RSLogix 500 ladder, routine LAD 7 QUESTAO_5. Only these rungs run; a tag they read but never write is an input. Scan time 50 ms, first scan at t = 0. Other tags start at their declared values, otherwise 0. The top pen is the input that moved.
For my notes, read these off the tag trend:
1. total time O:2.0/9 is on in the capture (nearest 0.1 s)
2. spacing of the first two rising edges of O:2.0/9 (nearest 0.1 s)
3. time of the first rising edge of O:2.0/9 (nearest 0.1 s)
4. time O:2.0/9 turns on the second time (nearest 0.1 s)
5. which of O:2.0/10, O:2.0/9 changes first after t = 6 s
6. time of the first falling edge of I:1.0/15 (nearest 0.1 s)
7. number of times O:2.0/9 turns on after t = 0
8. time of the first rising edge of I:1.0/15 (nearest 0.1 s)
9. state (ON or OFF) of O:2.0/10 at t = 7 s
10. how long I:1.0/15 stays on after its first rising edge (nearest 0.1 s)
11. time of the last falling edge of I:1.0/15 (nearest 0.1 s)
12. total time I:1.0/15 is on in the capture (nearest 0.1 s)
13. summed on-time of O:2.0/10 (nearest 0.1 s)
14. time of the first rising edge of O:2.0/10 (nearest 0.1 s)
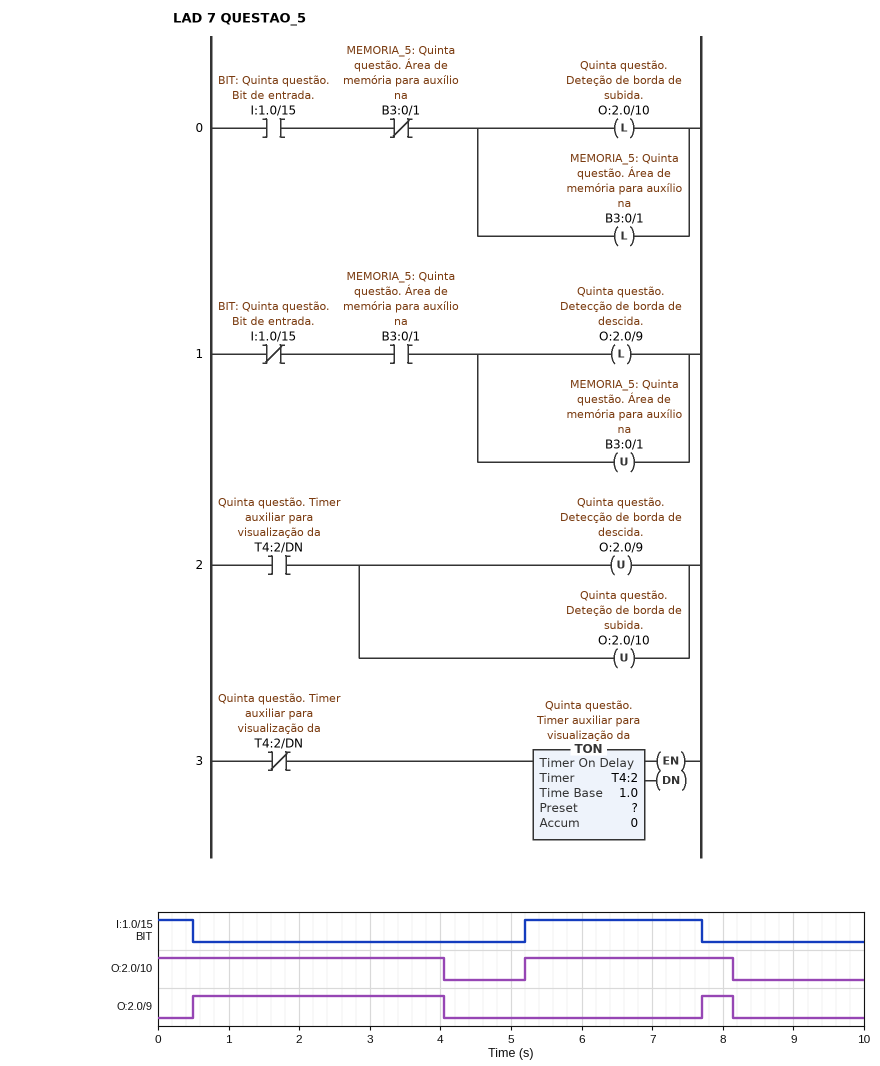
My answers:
4.0 s
7.2 s
0.5 s
7.7 s
O:2.0/9
0.5 s
2
5.2 s
ON
2.5 s
7.7 s
3.0 s
7.0 s
5.2 s
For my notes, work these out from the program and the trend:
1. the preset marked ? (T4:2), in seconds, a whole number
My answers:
4 s
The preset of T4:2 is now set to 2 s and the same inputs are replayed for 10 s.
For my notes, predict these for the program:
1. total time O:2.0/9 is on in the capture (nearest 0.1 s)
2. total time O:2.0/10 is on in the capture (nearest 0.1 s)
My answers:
2.2 s
3.1 s
